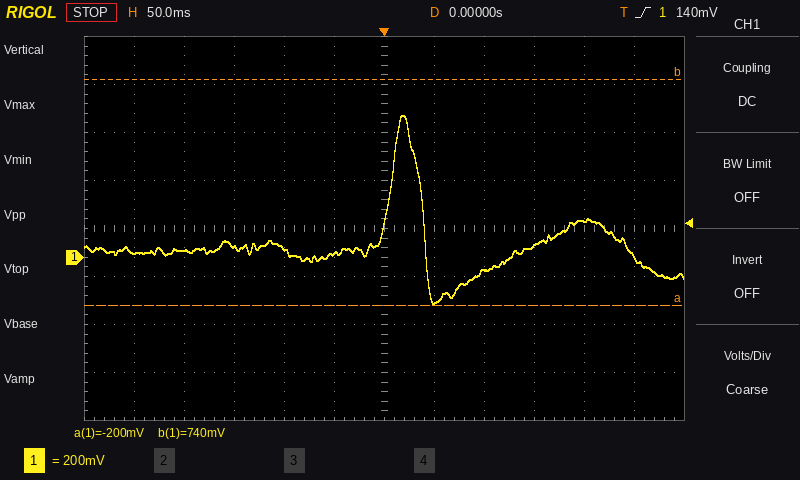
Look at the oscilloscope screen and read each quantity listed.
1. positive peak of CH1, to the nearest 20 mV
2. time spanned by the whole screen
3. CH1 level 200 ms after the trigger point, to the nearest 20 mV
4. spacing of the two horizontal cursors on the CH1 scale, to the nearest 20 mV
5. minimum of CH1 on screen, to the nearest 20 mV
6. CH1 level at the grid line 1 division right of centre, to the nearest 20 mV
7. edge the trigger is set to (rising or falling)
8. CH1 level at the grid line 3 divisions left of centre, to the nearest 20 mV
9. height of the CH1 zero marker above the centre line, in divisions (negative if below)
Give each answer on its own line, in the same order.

600 mV
600 ms
160 mV
940 mV
-200 mV
-180 mV
rising
40 mV
-0.6 div
